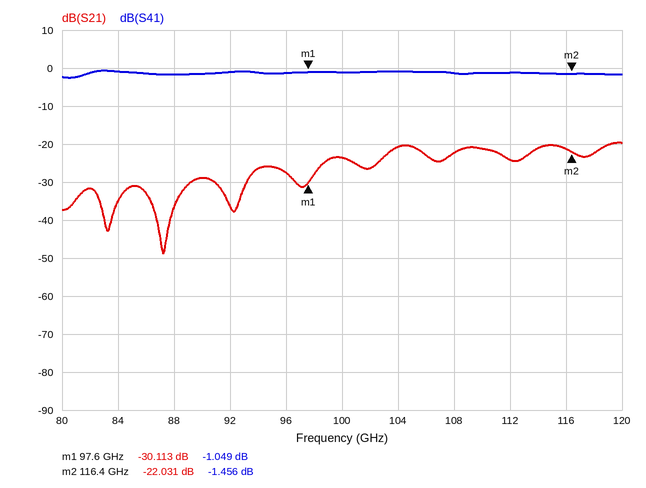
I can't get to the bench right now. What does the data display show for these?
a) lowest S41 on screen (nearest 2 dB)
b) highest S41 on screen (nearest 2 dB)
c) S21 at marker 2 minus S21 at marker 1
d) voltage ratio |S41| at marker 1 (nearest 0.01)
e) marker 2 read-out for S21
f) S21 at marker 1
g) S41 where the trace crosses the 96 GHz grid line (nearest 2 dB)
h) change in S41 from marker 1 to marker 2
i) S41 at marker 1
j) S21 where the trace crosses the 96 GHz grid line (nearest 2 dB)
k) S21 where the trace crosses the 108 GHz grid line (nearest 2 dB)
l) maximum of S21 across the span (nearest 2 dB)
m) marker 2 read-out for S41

-2 dB
0 dB
8.082 dB
0.89
-22.031 dB
-30.113 dB
-2 dB
-0.407 dB
-1.049 dB
-28 dB
-22 dB
-20 dB
-1.456 dB
